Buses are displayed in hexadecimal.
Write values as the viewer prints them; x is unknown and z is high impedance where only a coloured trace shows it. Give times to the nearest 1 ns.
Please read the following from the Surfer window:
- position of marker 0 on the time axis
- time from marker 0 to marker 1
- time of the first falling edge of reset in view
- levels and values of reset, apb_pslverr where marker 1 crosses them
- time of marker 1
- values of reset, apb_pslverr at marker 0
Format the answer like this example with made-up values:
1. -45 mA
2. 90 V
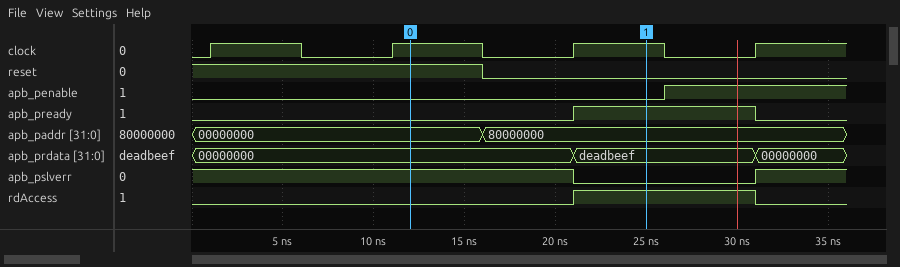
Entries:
1. 12 ns
2. 13 ns
3. 16 ns
4. reset=0, apb_pslverr=0
5. 25 ns
6. reset=1, apb_pslverr=1
